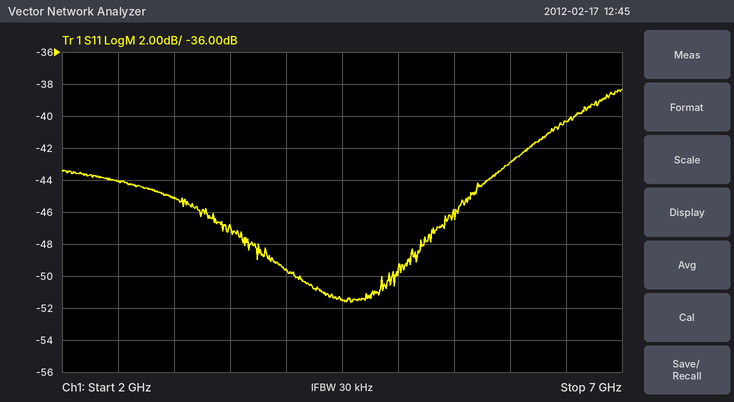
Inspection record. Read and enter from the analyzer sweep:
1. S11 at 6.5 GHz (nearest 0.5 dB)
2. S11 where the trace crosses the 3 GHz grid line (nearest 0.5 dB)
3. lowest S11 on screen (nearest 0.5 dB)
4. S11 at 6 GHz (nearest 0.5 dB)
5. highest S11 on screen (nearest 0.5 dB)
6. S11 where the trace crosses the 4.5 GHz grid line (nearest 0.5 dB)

-40.5 dB
-45.0 dB
-51.5 dB
-43.0 dB
-38.5 dB
-51.5 dB
